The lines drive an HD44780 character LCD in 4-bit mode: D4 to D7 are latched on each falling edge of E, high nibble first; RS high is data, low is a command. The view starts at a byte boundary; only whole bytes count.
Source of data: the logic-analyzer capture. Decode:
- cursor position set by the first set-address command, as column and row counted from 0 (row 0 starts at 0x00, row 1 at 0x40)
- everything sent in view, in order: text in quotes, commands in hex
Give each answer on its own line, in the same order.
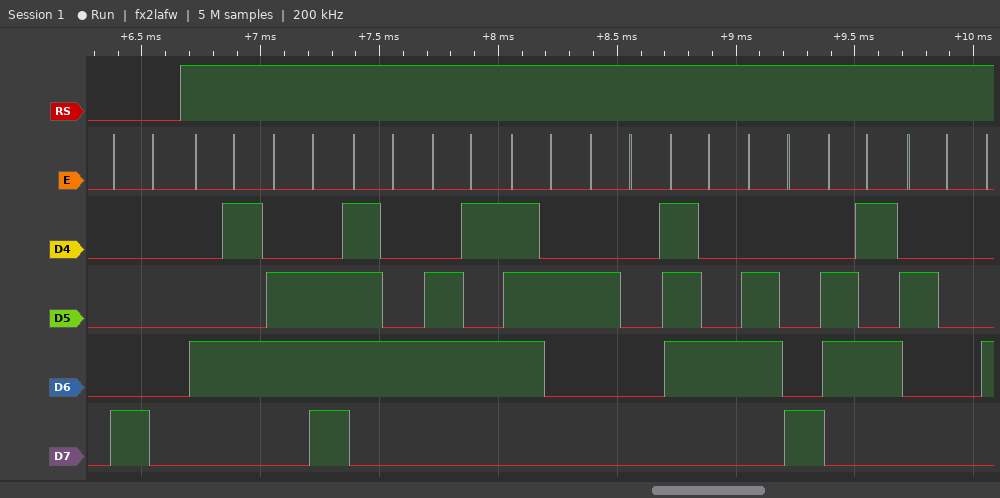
column 0, row 0
0x80 "Enter the "
